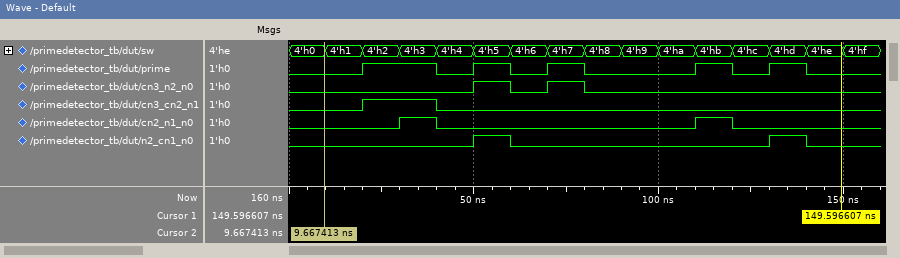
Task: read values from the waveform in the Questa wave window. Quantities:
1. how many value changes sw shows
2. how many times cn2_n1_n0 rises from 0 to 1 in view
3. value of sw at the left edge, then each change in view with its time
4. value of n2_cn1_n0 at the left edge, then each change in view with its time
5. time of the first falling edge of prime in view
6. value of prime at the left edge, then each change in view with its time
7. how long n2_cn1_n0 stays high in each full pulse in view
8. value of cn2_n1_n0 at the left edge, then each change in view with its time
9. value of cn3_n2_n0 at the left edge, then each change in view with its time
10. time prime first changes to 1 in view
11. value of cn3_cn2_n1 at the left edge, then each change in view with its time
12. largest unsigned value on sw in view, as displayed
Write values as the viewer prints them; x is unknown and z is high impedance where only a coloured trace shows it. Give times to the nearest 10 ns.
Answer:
15
2
4'h0, 4'h1 at 10 ns, 4'h2 at 20 ns, 4'h3 at 30 ns, 4'h4 at 40 ns, 4'h5 at 50 ns, 4'h6 at 60 ns, 4'h7 at 70 ns, 4'h8 at 80 ns, 4'h9 at 90 ns, 4'ha at 100 ns, 4'hb at 110 ns, 4'hc at 120 ns, 4'hd at 130 ns, 4'he at 140 ns, 4'hf at 150 ns
0, 1 at 50 ns, 0 at 60 ns, 1 at 130 ns, 0 at 140 ns
40 ns
0, 1 at 20 ns, 0 at 40 ns, 1 at 50 ns, 0 at 60 ns, 1 at 70 ns, 0 at 80 ns, 1 at 110 ns, 0 at 120 ns, 1 at 130 ns, 0 at 140 ns
10 ns, 10 ns
0, 1 at 30 ns, 0 at 40 ns, 1 at 110 ns, 0 at 120 ns
0, 1 at 50 ns, 0 at 60 ns, 1 at 70 ns, 0 at 80 ns
20 ns
0, 1 at 20 ns, 0 at 40 ns
4'hf
